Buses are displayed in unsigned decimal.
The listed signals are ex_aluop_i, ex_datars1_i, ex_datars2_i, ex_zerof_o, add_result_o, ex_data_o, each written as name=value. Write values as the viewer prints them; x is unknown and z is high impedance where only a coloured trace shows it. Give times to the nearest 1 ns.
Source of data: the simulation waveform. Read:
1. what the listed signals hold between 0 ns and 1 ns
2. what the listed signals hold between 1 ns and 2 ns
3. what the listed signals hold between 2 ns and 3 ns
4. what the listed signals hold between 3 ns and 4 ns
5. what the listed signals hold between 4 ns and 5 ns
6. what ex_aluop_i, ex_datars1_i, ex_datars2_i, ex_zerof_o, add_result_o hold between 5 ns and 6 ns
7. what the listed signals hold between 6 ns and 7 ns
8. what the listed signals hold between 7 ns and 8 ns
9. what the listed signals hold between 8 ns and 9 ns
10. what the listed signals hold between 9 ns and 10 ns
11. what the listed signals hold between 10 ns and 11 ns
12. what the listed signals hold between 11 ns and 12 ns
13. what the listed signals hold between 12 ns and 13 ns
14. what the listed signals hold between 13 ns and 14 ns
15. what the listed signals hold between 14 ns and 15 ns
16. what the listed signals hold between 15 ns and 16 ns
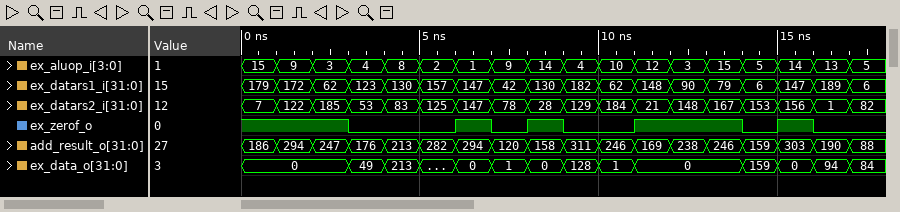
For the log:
ex_aluop_i=15, ex_datars1_i=179, ex_datars2_i=7, ex_zerof_o=1, add_result_o=186, ex_data_o=0
ex_aluop_i=9, ex_datars1_i=172, ex_datars2_i=122, ex_zerof_o=1, add_result_o=294, ex_data_o=0
ex_aluop_i=3, ex_datars1_i=62, ex_datars2_i=185, ex_zerof_o=1, add_result_o=247, ex_data_o=0
ex_aluop_i=4, ex_datars1_i=123, ex_datars2_i=53, ex_zerof_o=0, add_result_o=176, ex_data_o=49
ex_aluop_i=8, ex_datars1_i=130, ex_datars2_i=83, ex_zerof_o=0, add_result_o=213, ex_data_o=213
ex_aluop_i=2, ex_datars1_i=157, ex_datars2_i=125, ex_zerof_o=0, add_result_o=282
ex_aluop_i=1, ex_datars1_i=147, ex_datars2_i=147, ex_zerof_o=1, add_result_o=294, ex_data_o=0
ex_aluop_i=9, ex_datars1_i=42, ex_datars2_i=78, ex_zerof_o=0, add_result_o=120, ex_data_o=1
ex_aluop_i=14, ex_datars1_i=130, ex_datars2_i=28, ex_zerof_o=1, add_result_o=158, ex_data_o=0
ex_aluop_i=4, ex_datars1_i=182, ex_datars2_i=129, ex_zerof_o=0, add_result_o=311, ex_data_o=128
ex_aluop_i=10, ex_datars1_i=62, ex_datars2_i=184, ex_zerof_o=0, add_result_o=246, ex_data_o=1
ex_aluop_i=12, ex_datars1_i=148, ex_datars2_i=21, ex_zerof_o=1, add_result_o=169, ex_data_o=0
ex_aluop_i=3, ex_datars1_i=90, ex_datars2_i=148, ex_zerof_o=1, add_result_o=238, ex_data_o=0
ex_aluop_i=15, ex_datars1_i=79, ex_datars2_i=167, ex_zerof_o=1, add_result_o=246, ex_data_o=0
ex_aluop_i=5, ex_datars1_i=6, ex_datars2_i=153, ex_zerof_o=0, add_result_o=159, ex_data_o=159
ex_aluop_i=14, ex_datars1_i=147, ex_datars2_i=156, ex_zerof_o=1, add_result_o=303, ex_data_o=0
